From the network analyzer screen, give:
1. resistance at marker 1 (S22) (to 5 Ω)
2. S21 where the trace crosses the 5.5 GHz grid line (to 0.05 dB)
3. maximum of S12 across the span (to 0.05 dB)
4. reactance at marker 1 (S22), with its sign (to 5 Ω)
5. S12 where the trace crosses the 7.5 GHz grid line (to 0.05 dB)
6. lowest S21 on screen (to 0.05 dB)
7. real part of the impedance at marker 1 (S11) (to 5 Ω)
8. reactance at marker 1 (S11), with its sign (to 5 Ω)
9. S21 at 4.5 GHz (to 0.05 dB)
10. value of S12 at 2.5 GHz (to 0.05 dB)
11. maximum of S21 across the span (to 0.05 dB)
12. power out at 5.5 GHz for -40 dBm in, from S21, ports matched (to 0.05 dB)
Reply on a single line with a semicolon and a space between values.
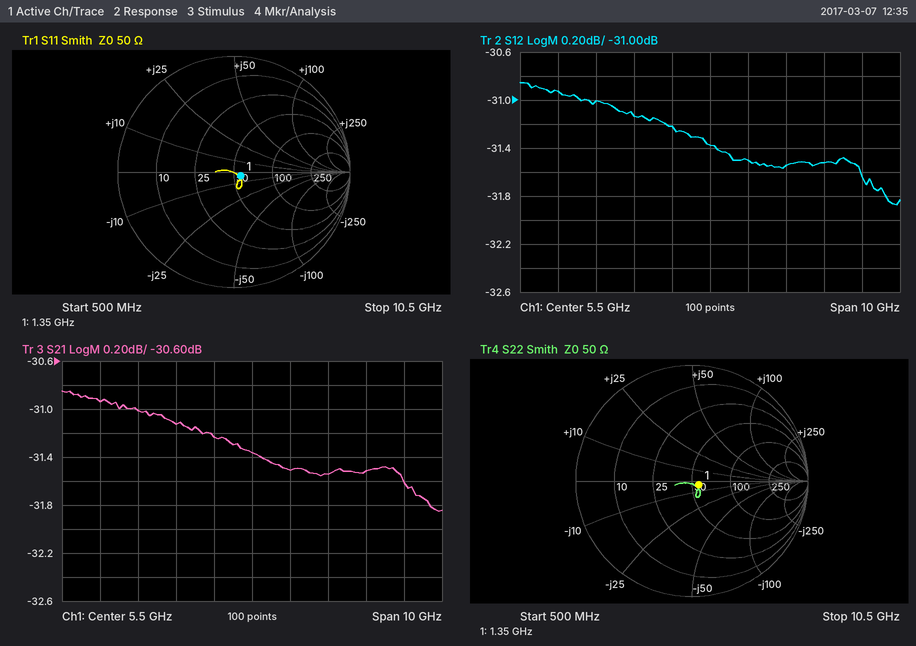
55 Ω; -31.35 dB; -30.85 dB; -5 Ω; -31.55 dB; -31.85 dB; 55 Ω; -5 Ω; -31.25 dB; -31.00 dB; -30.85 dB; -71.35 dBm
